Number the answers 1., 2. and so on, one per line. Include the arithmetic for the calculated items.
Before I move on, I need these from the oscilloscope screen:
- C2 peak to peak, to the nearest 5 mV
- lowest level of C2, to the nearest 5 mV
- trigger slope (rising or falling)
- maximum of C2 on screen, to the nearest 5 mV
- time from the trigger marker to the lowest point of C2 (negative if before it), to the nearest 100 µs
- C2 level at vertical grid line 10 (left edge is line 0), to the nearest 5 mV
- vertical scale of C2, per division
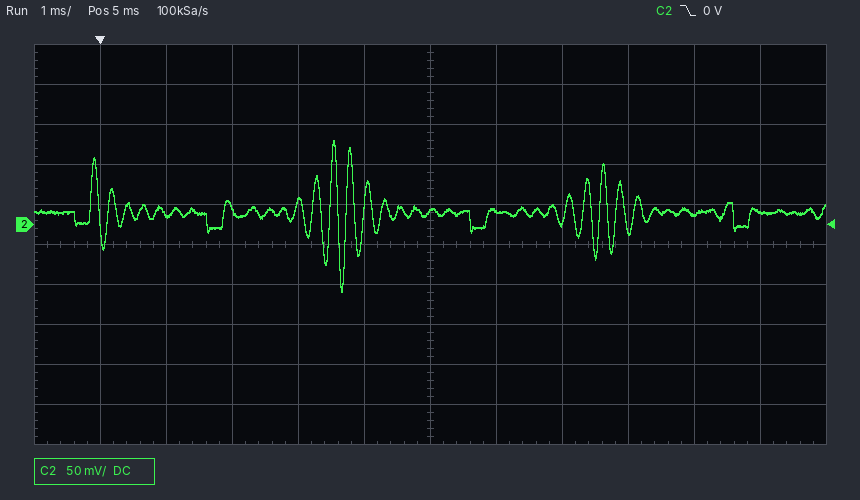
1. 105 mV − (-85 mV) = 190 mV
2. -85 mV
3. falling
4. 105 mV
5. +3.7 ms
6. 15 mV
7. 50 mV
